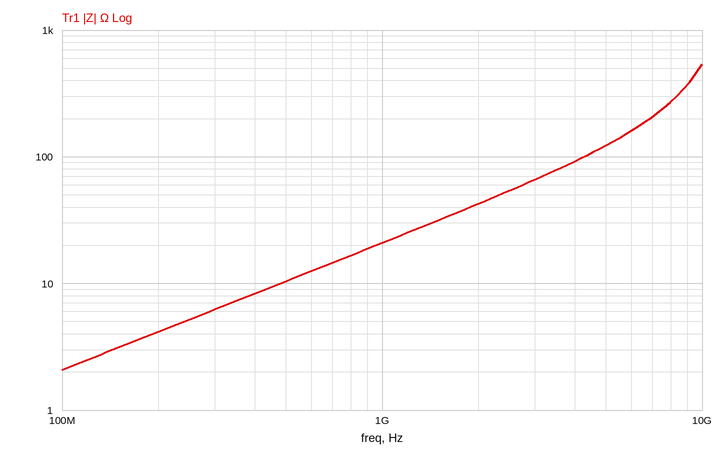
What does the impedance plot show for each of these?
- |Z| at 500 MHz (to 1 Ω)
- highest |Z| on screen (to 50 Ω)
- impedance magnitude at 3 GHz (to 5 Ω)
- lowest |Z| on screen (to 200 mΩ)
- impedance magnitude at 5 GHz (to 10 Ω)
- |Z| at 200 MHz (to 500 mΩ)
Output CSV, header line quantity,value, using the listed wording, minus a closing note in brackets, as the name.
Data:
quantity,value
|Z| at 500 MHz,10 Ω
highest |Z| on screen,550 Ω
impedance magnitude at 3 GHz,65 Ω
lowest |Z| on screen,2.0 Ω
impedance magnitude at 5 GHz,120 Ω
|Z| at 200 MHz,4.0 Ω
